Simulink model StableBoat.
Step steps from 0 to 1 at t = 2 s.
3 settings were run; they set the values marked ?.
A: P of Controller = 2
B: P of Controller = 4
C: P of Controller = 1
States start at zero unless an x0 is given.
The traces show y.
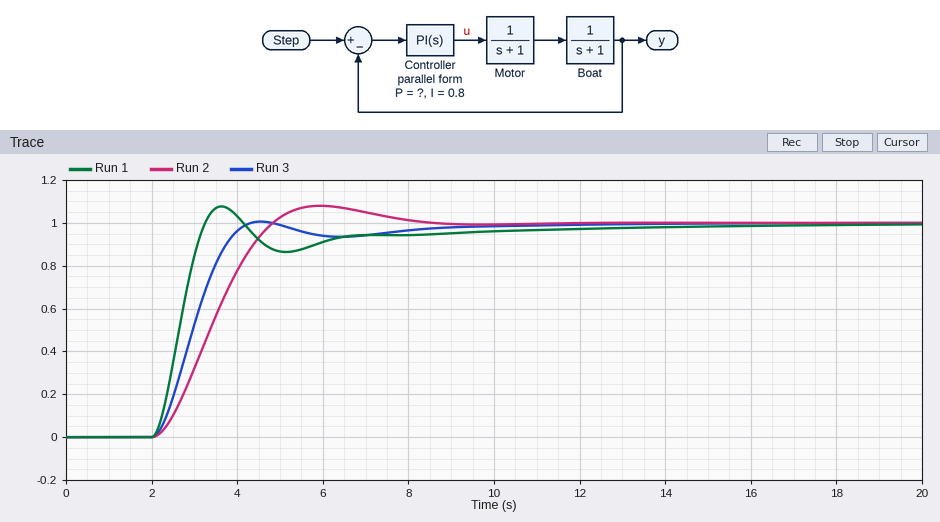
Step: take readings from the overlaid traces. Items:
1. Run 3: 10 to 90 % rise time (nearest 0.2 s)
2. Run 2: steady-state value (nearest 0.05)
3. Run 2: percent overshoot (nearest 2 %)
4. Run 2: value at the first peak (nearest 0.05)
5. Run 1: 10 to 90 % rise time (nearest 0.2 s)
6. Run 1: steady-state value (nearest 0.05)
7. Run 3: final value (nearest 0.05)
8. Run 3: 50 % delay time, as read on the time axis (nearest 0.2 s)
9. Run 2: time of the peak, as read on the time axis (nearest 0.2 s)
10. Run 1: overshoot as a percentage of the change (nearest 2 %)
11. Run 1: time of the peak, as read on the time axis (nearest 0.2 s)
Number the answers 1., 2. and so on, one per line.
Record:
1. 1.4 s
2. 1.00
3. 8 %
4. 1.10
5. 0.8 s
6. 1.00
7. 1.00
8. 3.0 s
9. 6.0 s
10. 8 %
11. 3.6 s
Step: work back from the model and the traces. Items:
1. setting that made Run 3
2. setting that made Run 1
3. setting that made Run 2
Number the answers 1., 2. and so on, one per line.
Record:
1. A
2. B
3. C
